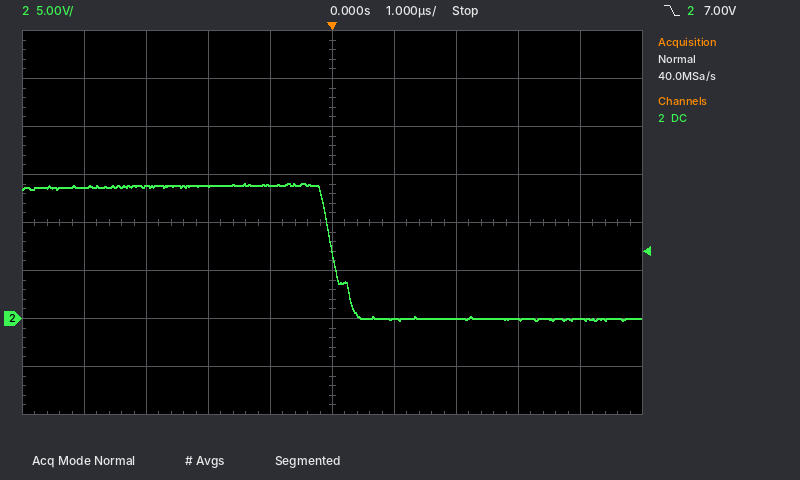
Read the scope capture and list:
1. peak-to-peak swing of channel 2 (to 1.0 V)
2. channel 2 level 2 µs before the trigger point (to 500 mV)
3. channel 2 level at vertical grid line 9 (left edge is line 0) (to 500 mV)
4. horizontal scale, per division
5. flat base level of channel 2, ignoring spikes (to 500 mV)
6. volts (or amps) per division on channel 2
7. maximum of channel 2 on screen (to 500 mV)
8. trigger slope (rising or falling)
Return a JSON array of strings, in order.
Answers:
["14.0 V", "14.0 V", "0.0 V", "1 µs", "0.0 V", "5 V", "14.0 V", "falling"]
